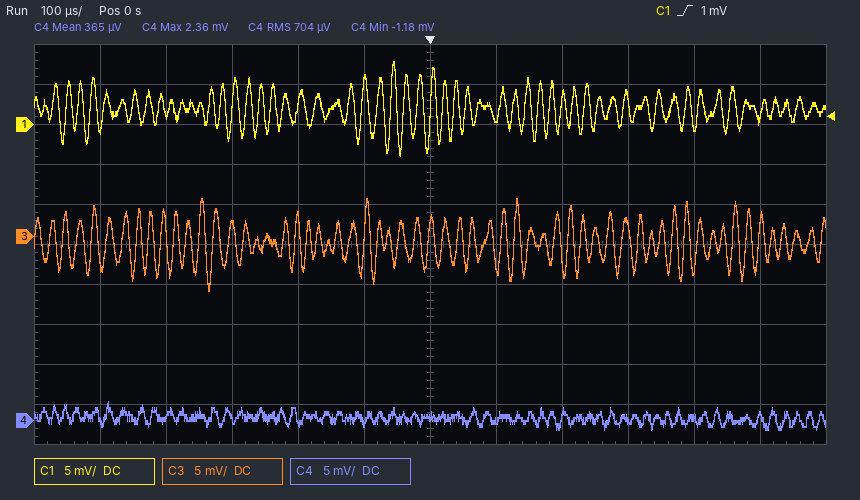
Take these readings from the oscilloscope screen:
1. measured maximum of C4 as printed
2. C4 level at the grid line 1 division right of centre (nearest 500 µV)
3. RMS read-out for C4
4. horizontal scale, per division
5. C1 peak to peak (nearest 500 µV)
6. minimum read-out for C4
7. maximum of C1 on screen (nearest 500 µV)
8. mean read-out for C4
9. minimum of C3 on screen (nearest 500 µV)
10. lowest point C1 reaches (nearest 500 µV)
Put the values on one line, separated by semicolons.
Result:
2.36 mV; 0.0 mV; 704 µV; 100 µs; 12.0 mV; -1.18 mV; 8.0 mV; 365 µV; -6.5 mV; -4.0 mV
